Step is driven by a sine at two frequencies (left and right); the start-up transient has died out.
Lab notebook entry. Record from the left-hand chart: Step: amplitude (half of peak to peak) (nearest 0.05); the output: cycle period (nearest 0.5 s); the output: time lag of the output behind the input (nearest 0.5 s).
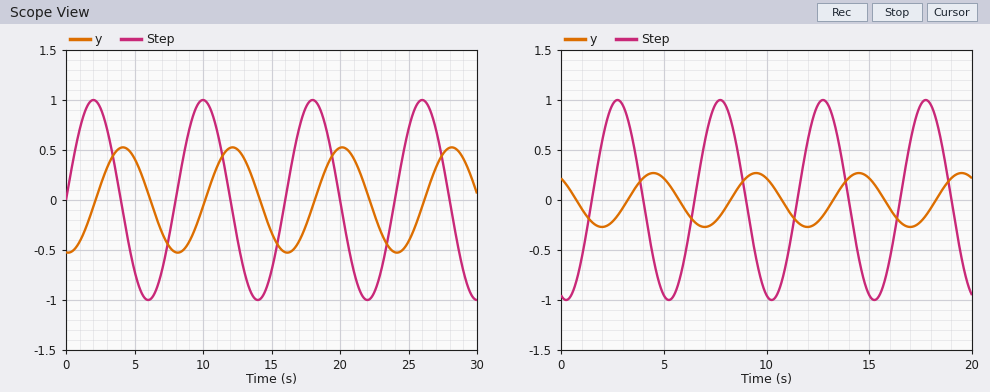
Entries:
1.00
8.0 s
2.0 s
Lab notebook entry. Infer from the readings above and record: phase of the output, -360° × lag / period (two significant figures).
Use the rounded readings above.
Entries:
-90°
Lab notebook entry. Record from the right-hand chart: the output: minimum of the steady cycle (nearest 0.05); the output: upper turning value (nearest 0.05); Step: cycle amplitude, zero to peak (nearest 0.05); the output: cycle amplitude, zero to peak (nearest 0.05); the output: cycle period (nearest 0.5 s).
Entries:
-0.25
0.25
1.00
0.25
5.0 s
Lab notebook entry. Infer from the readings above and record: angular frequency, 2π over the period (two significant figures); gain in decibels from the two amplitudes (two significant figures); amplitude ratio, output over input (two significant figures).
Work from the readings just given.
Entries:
1.3 rad/s
-12 dB
0.25
